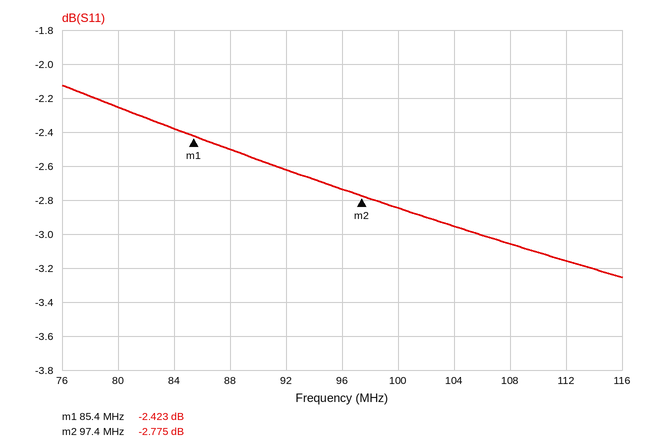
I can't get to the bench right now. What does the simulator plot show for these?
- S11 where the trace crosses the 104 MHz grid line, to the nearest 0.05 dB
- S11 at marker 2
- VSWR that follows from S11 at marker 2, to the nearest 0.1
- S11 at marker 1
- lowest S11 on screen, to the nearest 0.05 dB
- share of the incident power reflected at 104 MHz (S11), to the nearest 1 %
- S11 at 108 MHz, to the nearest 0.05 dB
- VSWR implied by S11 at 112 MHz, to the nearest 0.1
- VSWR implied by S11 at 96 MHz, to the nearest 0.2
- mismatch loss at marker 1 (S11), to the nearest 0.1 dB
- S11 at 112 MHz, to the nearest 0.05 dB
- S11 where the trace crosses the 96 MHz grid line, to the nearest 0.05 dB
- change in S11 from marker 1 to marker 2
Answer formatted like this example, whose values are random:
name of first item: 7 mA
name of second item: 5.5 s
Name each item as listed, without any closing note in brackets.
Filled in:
S11 where the trace crosses the 104 MHz grid line, to the nearest 0.05 dB: -2.95 dB
S11 at marker 2: -2.775 dB
VSWR that follows from S11 at marker 2, to the nearest 0.1: 6.3
S11 at marker 1: -2.423 dB
lowest S11 on screen, to the nearest 0.05 dB: -3.25 dB
share of the incident power reflected at 104 MHz (S11), to the nearest 1 %: 51 %
S11 at 108 MHz, to the nearest 0.05 dB: -3.05 dB
VSWR implied by S11 at 112 MHz, to the nearest 0.1: 5.6
VSWR implied by S11 at 96 MHz, to the nearest 0.2: 6.4
mismatch loss at marker 1 (S11), to the nearest 0.1 dB: 3.7 dB
S11 at 112 MHz, to the nearest 0.05 dB: -3.15 dB
S11 where the trace crosses the 96 MHz grid line, to the nearest 0.05 dB: -2.75 dB
change in S11 from marker 1 to marker 2: -0.352 dB
